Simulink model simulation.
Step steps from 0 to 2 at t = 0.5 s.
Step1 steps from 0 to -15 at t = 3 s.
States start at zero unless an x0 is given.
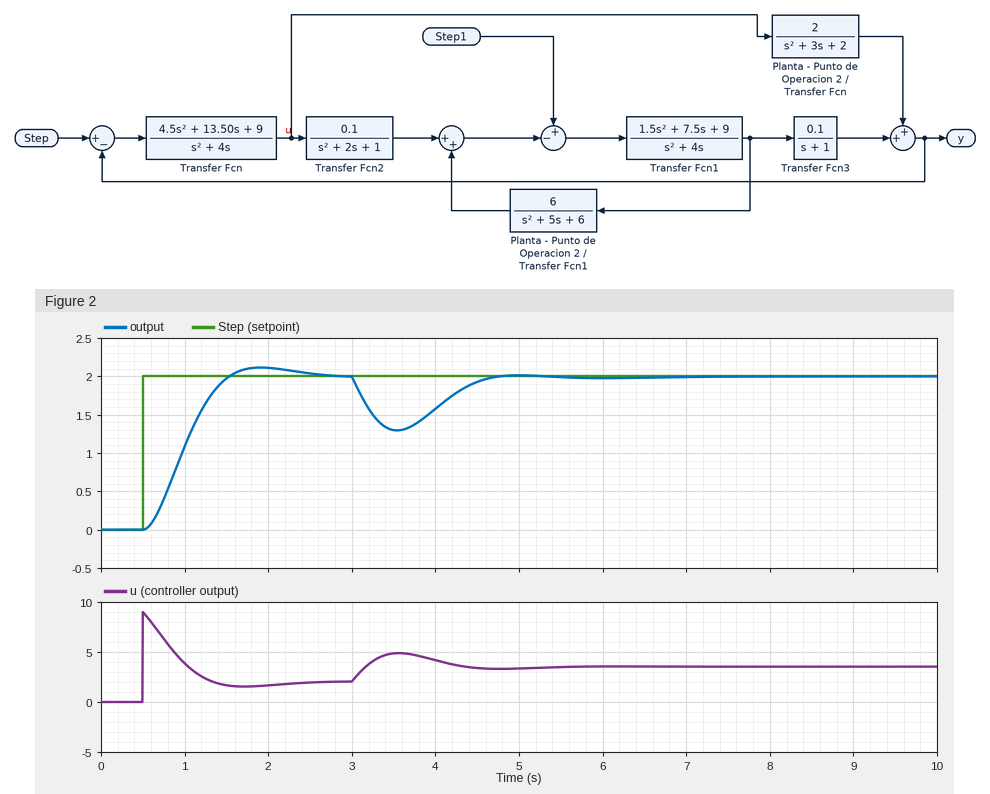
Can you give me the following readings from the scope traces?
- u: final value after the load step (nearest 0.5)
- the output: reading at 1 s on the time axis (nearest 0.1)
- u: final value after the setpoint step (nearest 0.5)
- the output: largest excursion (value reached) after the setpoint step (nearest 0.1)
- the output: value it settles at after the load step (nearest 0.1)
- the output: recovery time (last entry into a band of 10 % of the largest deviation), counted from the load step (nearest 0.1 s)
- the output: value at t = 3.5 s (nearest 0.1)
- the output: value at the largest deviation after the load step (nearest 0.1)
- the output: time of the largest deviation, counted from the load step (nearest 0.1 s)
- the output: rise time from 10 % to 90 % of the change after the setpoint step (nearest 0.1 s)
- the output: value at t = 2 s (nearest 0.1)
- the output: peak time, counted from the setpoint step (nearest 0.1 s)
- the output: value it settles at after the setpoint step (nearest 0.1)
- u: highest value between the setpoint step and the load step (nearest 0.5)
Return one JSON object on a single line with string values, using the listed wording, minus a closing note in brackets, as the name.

{"u: final value after the load step": "3.5", "the output: reading at 1 s on the time axis": "1.1", "u: final value after the setpoint step": "2.0", "the output: largest excursion (value reached) after the setpoint step": "2.1", "the output: value it settles at after the load step": "2.0", "the output: recovery time (last entry into a band of 10 % of the largest deviation), counted from the load step": "1.5 s", "the output: value at t = 3.5 s": "1.3", "the output: value at the largest deviation after the load step": "1.3", "the output: time of the largest deviation, counted from the load step": "0.5 s", "the output: rise time from 10 % to 90 % of the change after the setpoint step": "0.7 s", "the output: value at t = 2 s": "2.1", "the output: peak time, counted from the setpoint step": "1.4 s", "the output: value it settles at after the setpoint step": "2.0", "u: highest value between the setpoint step and the load step": "9.0"}
